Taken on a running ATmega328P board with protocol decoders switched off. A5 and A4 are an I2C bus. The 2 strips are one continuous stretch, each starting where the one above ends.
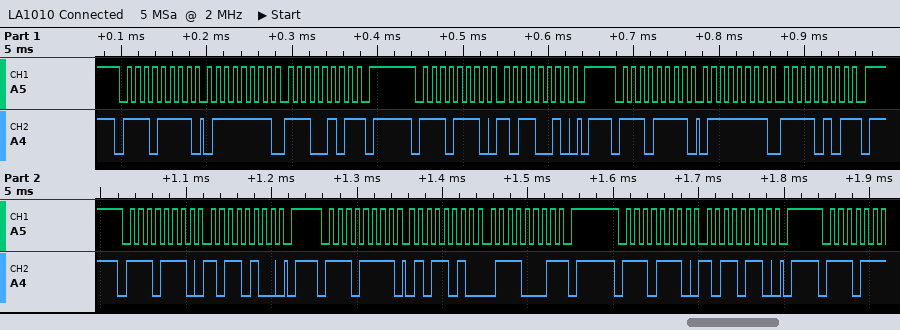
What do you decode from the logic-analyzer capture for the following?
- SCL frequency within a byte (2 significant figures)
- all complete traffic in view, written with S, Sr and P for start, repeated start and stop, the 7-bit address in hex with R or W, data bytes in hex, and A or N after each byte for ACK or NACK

100 kHz
S 77R A 7F A E5 N P S 77W A B2 A P S 77R A 7F A F5 N P S 77W A B4 A P S 77R A 5A A 71 N P S 77W A B6 A P
